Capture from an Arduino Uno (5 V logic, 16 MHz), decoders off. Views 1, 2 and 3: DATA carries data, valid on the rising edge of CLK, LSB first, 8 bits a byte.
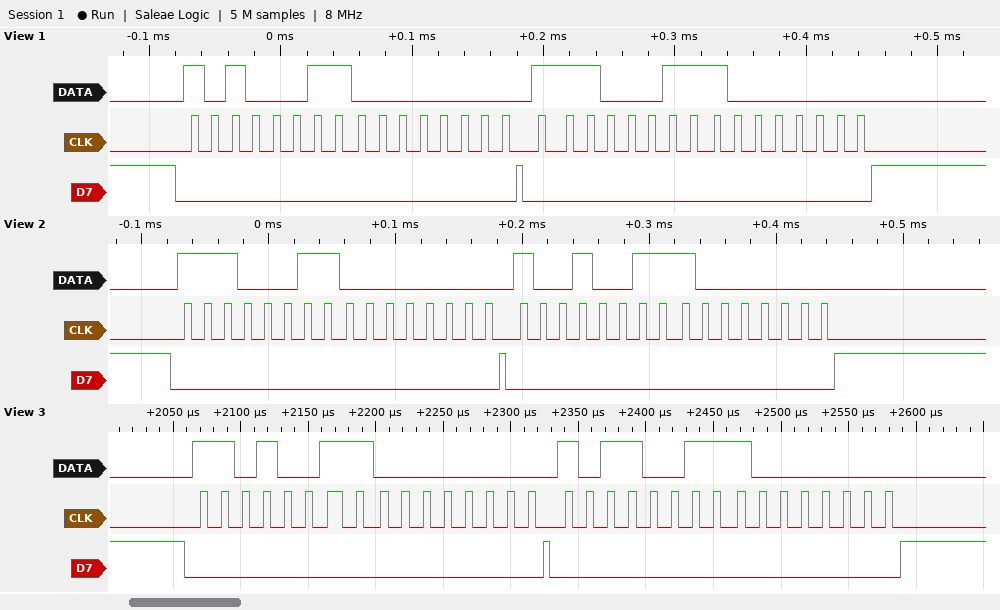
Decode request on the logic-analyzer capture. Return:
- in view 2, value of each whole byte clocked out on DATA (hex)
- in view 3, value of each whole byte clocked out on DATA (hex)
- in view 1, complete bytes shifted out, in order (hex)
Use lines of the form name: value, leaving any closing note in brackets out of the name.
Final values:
in view 2, value of each whole byte clocked out on DATA: C7 00 C9 01
in view 3, value of each whole byte clocked out on DATA: CB 00 CD 01
in view 1, complete bytes shifted out, in order: 0xC5 0x00 0xC7 0x01
